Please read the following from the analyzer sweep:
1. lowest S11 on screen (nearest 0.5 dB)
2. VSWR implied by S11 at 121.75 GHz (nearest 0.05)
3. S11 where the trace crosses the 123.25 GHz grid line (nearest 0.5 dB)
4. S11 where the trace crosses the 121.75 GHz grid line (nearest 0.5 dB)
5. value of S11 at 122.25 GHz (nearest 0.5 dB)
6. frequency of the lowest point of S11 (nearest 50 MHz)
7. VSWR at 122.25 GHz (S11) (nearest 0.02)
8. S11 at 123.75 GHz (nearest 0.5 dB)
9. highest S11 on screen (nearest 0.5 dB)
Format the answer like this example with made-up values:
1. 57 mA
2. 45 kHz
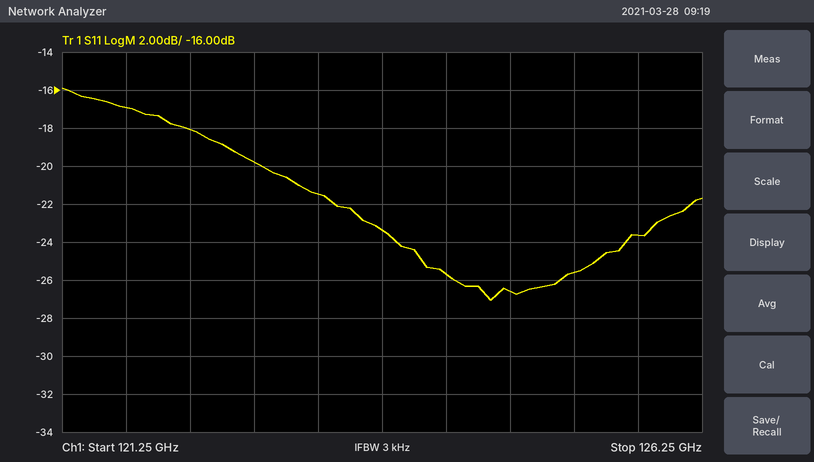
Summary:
1. -27.0 dB
2. 1.35
3. -21.5 dB
4. -17.0 dB
5. -18.0 dB
6. 124.60 GHz
7. 1.28
8. -23.5 dB
9. -16.0 dB
